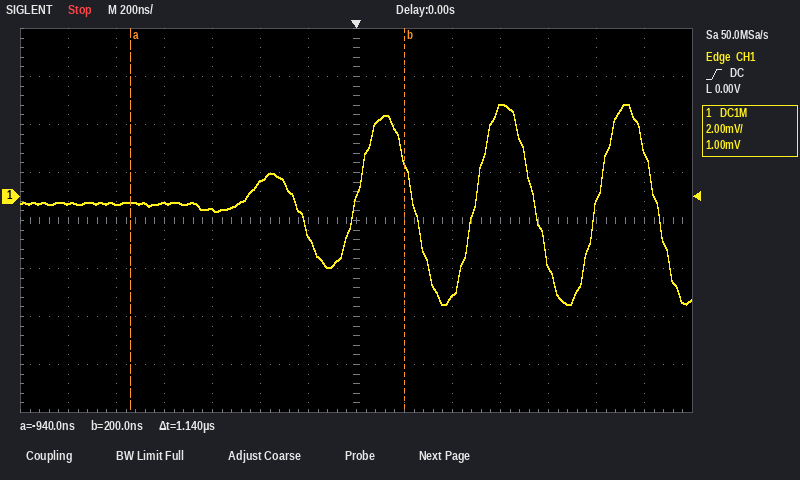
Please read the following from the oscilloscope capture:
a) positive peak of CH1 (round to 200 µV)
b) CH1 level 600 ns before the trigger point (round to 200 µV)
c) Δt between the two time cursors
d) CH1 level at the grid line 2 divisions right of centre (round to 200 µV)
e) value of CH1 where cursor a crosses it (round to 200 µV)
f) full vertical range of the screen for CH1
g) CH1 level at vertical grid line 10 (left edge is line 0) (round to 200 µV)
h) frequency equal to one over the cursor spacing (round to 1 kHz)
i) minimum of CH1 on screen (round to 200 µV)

3.8 mV
-600 µV
1.14 µs
-4.2 mV
-200 µV
16 mV
3.8 mV
877 kHz
-4.4 mV
